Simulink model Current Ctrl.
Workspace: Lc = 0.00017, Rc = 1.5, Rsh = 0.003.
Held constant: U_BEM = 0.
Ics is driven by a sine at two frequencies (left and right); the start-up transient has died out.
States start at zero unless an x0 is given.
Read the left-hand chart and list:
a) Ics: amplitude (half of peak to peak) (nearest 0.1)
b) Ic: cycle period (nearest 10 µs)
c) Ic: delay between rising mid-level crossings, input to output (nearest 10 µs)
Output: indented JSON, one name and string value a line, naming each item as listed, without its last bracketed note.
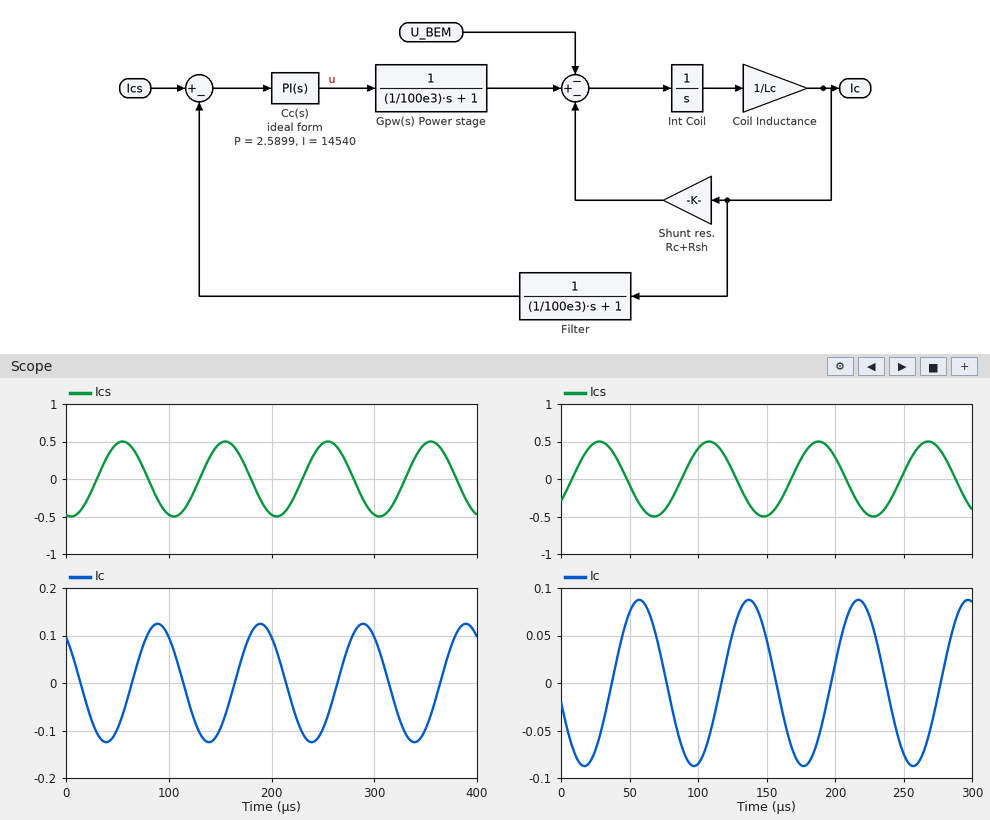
{
  "Ics: amplitude (half of peak to peak)": "0.5",
  "Ic: cycle period": "100 µs",
  "Ic: delay between rising mid-level crossings, input to output": "30 µs"
}
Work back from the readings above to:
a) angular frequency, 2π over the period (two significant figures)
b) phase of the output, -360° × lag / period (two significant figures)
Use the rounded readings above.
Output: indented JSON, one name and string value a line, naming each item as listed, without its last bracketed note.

{
  "angular frequency, 2π over the period": "0.063 rad/µs",
  "phase of the output, -360° × lag / period": "-110°"
}
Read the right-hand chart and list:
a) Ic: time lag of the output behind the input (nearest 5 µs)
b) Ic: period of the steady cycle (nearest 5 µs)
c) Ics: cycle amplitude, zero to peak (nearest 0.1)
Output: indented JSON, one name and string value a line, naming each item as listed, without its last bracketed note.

{
  "Ic: time lag of the output behind the input": "30 µs",
  "Ic: period of the steady cycle": "80 µs",
  "Ics: cycle amplitude, zero to peak": "0.5"
}
